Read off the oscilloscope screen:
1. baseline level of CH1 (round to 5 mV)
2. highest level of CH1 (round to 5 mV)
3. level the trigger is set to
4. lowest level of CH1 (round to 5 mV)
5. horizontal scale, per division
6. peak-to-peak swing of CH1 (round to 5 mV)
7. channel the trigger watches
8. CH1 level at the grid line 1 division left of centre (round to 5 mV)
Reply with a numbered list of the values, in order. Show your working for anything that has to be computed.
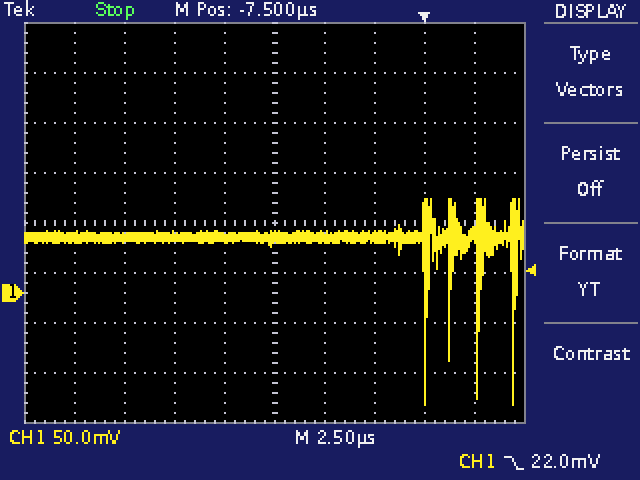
1. 55 mV
2. 95 mV
3. 22.0 mV
4. -110 mV
5. 2.5 µs
6. 95 mV − (-110 mV) = 205 mV
7. CH1
8. 55 mV
